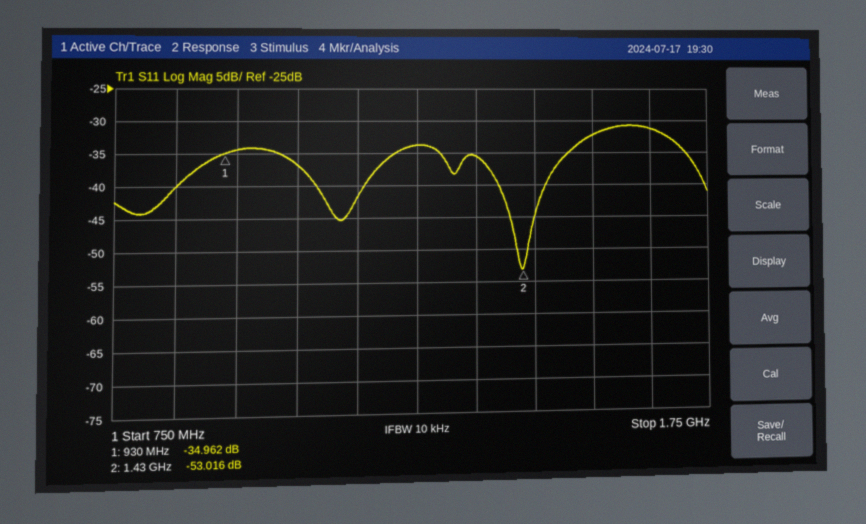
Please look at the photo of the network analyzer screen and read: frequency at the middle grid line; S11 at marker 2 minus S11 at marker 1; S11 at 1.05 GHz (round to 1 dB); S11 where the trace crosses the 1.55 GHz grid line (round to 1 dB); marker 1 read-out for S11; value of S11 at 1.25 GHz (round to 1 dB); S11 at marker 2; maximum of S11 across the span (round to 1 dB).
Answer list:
1.25 GHz
-18.054 dB
-37 dB
-32 dB
-34.962 dB
-34 dB
-53.016 dB
-31 dB
